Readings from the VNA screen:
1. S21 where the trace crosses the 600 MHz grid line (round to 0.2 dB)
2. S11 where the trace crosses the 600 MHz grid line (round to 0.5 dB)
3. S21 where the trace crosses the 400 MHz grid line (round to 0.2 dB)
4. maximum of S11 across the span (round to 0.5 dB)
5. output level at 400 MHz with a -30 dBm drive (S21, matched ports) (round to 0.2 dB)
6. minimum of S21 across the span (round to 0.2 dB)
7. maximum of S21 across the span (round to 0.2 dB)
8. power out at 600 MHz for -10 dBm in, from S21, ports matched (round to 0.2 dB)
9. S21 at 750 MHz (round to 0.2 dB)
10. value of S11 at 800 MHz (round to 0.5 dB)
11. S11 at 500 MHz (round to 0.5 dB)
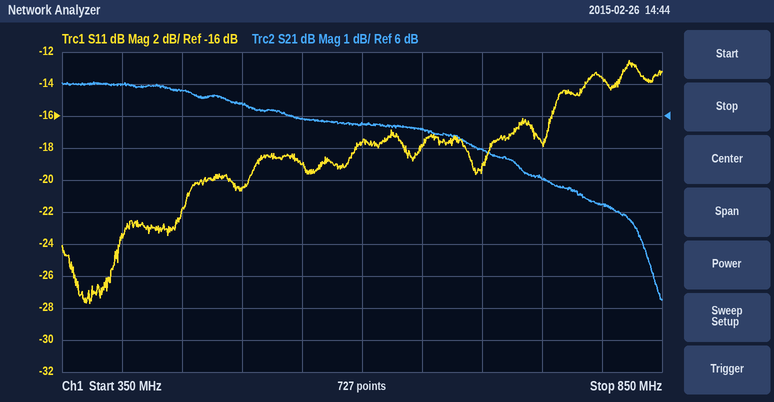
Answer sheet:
5.8 dB
-17.5 dB
7.0 dB
-12.5 dB
-23.0 dBm
0.2 dB
7.0 dB
-4.2 dBm
4.0 dB
-13.5 dB
-20.5 dB
